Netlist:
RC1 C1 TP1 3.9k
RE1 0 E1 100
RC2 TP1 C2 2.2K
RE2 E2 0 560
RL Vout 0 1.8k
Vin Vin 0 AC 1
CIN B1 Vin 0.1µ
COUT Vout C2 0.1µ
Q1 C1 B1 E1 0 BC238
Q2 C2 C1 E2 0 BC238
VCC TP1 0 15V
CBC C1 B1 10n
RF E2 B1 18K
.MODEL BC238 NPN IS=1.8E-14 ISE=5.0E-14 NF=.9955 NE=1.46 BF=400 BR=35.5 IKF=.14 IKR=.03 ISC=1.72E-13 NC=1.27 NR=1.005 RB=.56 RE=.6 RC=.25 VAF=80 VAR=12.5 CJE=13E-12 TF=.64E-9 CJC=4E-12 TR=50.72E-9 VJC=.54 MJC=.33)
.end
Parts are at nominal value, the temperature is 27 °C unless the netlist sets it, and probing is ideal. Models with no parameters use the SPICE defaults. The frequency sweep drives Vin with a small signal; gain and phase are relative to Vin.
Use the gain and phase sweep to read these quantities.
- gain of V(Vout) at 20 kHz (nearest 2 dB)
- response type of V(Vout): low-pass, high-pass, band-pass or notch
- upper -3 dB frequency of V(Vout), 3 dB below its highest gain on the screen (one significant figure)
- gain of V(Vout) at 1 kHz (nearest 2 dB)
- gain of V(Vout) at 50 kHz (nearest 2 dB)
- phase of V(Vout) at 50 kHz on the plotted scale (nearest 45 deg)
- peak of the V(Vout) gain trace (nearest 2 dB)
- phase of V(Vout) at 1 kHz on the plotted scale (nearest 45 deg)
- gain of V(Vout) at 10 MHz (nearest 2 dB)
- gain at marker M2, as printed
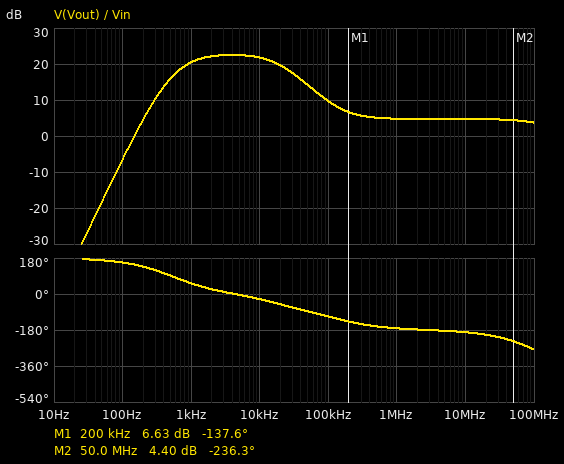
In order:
20 dB
band-pass
20 kHz
20 dB
14 dB
-90 deg
22 dB
45 deg
4 dB
4.40 dB
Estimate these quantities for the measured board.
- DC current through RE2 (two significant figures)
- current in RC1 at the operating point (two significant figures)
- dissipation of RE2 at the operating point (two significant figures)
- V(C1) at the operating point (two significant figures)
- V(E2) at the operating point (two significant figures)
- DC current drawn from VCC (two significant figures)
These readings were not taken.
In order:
2.2 mA
3.4 mA
2.6 mW
1.9 V
1.2 V
5.5 mA
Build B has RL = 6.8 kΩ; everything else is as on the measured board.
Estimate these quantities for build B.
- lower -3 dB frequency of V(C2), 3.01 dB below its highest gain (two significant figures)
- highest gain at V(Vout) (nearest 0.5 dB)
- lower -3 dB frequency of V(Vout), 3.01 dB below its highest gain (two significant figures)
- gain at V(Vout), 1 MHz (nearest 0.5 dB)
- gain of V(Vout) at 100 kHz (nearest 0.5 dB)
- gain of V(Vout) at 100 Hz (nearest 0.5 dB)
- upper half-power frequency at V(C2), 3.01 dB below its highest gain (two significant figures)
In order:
630 Hz
27.0 dB
700 Hz
9.5 dB
14.0 dB
4.0 dB
20 kHz
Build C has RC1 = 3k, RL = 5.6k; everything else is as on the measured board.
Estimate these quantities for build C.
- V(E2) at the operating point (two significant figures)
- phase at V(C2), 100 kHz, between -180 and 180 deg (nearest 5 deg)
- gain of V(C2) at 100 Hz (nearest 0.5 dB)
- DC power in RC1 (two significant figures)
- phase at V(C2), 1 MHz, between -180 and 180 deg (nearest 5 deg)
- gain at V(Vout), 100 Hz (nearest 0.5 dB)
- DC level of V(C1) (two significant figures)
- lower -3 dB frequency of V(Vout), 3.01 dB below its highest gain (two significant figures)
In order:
1.4 V
-110 deg
12.0 dB
56 mW
-170 deg
2.5 dB
2.0 V
690 Hz
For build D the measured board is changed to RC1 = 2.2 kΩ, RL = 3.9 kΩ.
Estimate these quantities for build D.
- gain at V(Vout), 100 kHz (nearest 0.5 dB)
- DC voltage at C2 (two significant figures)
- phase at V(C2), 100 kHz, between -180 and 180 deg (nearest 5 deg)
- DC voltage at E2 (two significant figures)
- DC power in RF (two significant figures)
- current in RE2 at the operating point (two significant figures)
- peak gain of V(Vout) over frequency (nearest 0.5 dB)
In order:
13.0 dB
8.6 V
-110 deg
1.6 V
6.8 µW
2.9 mA
24.5 dB
